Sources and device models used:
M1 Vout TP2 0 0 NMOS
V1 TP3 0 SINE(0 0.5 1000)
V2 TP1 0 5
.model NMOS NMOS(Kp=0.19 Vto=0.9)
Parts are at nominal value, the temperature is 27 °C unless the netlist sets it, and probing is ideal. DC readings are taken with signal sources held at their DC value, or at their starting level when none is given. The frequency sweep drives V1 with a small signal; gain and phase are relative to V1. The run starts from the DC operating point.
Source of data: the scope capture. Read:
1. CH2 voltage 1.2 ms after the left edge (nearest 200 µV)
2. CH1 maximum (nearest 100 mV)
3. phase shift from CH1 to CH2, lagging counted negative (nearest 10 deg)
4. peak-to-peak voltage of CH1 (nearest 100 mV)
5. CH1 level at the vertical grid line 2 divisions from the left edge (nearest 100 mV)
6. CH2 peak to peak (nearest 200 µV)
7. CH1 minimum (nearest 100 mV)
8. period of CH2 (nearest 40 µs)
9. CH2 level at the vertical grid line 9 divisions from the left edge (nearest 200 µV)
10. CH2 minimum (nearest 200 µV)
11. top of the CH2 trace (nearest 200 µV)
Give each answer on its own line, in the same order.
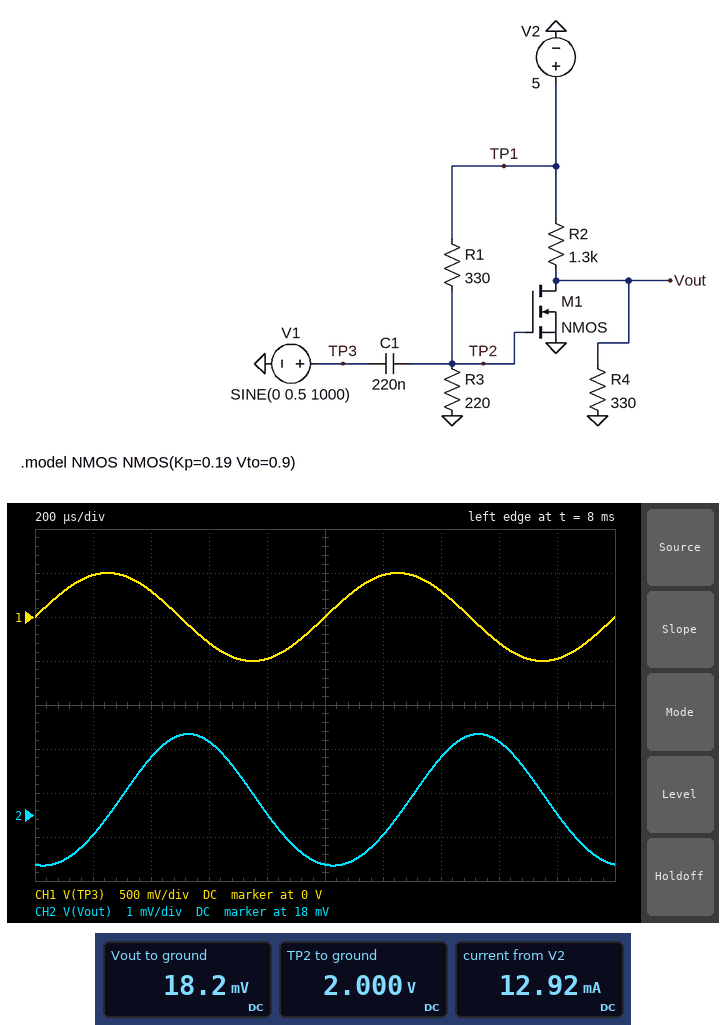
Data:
17.6 mV
500 mV
-100 deg
1.0 V
300 mV
3.0 mV
-500 mV
1.00 ms
18.0 mV
16.8 mV
19.8 mV
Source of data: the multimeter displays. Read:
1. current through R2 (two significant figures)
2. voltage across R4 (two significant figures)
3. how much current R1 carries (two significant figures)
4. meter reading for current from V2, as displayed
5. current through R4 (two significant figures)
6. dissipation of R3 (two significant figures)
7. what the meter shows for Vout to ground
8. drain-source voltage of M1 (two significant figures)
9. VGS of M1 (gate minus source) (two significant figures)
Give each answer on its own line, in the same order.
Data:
3.8 mA
18 mV
9.1 mA
12.92 mA
55 µA
18 mW
18.2 mV
18 mV
2.0 V
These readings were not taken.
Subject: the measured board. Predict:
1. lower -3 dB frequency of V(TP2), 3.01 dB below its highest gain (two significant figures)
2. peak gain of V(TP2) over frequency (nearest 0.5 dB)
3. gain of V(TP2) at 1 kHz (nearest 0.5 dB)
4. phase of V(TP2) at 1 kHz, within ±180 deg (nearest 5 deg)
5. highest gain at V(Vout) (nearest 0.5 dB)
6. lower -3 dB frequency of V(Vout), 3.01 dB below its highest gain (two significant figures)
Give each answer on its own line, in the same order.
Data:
5.5 kHz
0 dB
-15.0 dB
80 deg
-35.5 dB
5.5 kHz
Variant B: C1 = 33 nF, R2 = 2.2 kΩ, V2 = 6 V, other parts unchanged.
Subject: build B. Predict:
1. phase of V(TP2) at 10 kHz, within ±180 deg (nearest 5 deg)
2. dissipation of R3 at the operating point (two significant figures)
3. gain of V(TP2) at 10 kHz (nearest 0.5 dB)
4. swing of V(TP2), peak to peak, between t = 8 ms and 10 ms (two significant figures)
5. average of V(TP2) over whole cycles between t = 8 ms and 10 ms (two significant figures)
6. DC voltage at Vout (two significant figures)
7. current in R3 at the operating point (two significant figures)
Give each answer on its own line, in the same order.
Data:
75 deg
26 mW
-11.5 dB
27 mV
2.4 V
9.5 mV
11 mA
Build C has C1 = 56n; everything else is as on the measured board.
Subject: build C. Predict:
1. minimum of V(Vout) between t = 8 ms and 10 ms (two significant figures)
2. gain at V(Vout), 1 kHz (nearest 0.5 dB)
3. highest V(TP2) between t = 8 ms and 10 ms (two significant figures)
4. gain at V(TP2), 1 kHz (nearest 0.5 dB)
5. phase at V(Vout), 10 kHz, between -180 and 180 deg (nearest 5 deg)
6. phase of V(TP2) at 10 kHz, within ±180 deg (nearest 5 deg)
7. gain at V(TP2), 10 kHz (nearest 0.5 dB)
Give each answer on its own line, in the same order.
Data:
18 mV
-62.5 dB
2.0 V
-26.5 dB
-115 deg
65 deg
-7.5 dB
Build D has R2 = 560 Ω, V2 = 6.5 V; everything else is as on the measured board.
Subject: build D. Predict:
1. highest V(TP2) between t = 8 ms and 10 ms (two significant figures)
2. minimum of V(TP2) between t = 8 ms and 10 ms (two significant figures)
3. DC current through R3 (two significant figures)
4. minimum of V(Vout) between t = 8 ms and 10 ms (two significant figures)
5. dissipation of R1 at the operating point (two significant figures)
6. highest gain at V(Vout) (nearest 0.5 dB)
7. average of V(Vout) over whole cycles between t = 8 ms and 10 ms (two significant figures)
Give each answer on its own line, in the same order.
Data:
2.7 V
2.5 V
12 mA
34 mV
46 mW
-33.5 dB
36 mV
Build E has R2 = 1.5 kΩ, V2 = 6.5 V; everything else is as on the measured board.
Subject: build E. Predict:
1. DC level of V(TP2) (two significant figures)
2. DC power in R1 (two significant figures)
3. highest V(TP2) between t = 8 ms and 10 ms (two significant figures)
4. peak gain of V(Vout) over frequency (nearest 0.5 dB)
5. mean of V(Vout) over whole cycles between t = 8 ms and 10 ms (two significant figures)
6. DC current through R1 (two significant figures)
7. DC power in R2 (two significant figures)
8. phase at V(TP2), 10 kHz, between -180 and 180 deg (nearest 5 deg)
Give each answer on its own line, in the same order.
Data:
2.6 V
46 mW
2.7 V
-42.0 dB
13 mV
12 mA
28 mW
30 deg
